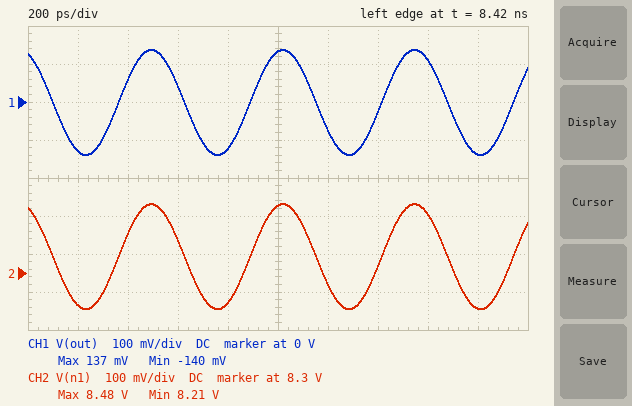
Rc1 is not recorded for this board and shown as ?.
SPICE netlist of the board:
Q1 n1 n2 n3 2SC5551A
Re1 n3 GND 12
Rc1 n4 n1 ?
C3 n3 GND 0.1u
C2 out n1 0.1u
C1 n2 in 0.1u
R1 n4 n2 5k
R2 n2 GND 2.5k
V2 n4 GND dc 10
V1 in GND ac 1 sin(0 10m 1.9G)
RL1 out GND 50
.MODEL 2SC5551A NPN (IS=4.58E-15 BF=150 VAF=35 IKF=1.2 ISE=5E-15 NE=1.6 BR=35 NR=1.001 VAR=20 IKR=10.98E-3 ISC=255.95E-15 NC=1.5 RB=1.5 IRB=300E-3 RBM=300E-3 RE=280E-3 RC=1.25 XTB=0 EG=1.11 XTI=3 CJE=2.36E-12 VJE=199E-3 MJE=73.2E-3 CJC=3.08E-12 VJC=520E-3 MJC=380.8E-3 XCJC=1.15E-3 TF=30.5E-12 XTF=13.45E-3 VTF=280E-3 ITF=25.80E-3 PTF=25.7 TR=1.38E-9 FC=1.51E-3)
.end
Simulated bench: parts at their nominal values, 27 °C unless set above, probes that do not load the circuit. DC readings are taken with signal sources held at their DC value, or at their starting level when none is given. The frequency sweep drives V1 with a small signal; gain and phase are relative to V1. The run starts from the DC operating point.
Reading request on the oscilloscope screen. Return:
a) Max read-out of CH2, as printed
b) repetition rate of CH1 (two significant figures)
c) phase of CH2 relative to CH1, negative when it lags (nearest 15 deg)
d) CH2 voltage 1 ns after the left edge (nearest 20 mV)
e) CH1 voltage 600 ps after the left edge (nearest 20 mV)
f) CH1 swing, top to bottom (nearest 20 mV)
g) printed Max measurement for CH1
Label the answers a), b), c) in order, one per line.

a) 8.48 V
b) 1.9 GHz
c) 0 deg
d) 8.48 V
e) 40 mV
f) 280 mV
g) 137 mV
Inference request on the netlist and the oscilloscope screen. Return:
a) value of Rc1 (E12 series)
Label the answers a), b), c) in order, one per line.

a) 15 Ω
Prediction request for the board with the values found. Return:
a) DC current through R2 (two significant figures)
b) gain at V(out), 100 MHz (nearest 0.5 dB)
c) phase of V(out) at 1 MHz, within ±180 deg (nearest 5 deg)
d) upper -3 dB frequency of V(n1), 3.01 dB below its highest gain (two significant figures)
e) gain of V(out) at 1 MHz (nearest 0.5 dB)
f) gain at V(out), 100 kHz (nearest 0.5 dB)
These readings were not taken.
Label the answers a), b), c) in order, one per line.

a) 860 µA
b) 26.5 dB
c) -115 deg
d) 1.7 GHz
e) 16.5 dB
f) 1.0 dB
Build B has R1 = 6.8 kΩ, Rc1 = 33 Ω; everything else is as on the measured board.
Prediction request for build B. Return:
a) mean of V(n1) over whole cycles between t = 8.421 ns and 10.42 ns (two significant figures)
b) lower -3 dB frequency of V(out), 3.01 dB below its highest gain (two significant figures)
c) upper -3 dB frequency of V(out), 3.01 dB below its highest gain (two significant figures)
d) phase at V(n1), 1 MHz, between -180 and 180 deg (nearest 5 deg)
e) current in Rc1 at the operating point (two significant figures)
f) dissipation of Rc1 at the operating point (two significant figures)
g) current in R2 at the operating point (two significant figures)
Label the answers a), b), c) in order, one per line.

a) 7.4 V
b) 2.6 MHz
c) 1.9 GHz
d) -120 deg
e) 79 mA
f) 210 mW
g) 710 µA
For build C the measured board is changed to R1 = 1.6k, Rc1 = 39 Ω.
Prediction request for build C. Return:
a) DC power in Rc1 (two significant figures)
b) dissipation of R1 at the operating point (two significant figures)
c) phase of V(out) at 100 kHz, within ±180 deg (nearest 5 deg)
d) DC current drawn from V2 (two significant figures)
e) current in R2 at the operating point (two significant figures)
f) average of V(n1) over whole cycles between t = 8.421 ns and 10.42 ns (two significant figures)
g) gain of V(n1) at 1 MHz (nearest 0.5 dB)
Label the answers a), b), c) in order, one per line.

a) 1.4 W
b) 29 mW
c) -70 deg
d) 190 mA
e) 1.3 mA
f) 2.7 V
g) 2.5 dB
